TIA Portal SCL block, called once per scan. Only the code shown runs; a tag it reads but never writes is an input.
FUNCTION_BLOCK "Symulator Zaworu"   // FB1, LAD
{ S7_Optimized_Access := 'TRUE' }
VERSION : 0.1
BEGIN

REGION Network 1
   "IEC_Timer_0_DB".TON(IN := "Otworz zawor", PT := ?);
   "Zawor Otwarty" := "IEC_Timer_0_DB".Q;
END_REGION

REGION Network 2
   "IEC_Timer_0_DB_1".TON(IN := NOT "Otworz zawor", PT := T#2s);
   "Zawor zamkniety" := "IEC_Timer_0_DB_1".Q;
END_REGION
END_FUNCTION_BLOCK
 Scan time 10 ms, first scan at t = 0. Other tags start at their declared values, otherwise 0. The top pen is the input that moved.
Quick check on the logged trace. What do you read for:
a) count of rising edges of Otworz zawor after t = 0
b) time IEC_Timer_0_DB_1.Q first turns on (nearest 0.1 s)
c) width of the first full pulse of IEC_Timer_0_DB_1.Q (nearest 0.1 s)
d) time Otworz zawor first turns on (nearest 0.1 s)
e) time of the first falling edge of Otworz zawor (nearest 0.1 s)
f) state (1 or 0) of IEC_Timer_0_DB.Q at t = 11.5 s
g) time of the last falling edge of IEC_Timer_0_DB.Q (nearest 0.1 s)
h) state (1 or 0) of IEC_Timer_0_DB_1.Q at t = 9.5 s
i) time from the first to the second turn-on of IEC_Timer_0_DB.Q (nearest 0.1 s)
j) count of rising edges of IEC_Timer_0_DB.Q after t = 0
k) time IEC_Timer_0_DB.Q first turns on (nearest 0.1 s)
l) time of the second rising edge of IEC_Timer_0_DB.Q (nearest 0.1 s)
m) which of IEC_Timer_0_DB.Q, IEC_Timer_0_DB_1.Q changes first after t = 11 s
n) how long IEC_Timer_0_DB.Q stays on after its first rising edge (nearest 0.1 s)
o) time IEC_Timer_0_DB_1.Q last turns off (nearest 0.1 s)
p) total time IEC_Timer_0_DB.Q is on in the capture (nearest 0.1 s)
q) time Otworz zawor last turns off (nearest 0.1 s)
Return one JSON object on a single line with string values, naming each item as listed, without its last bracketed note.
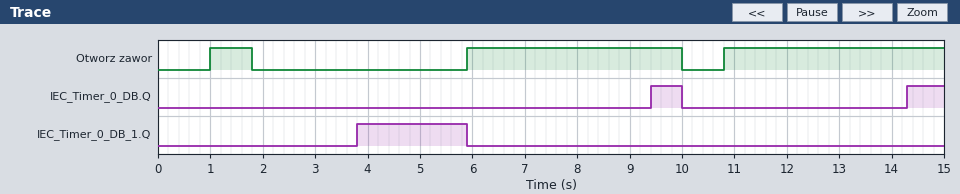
{"count of rising edges of Otworz zawor after t = 0": "3", "time IEC_Timer_0_DB_1.Q first turns on": "3.8 s", "width of the first full pulse of IEC_Timer_0_DB_1.Q": "2.1 s", "time Otworz zawor first turns on": "1.0 s", "time of the first falling edge of Otworz zawor": "1.8 s", "state (1 or 0) of IEC_Timer_0_DB.Q at t = 11.5 s": "0", "time of the last falling edge of IEC_Timer_0_DB.Q": "10.0 s", "state (1 or 0) of IEC_Timer_0_DB_1.Q at t = 9.5 s": "0", "time from the first to the second turn-on of IEC_Timer_0_DB.Q": "4.9 s", "count of rising edges of IEC_Timer_0_DB.Q after t = 0": "2", "time IEC_Timer_0_DB.Q first turns on": "9.4 s", "time of the second rising edge of IEC_Timer_0_DB.Q": "14.3 s", "which of IEC_Timer_0_DB.Q, IEC_Timer_0_DB_1.Q changes first after t = 11 s": "IEC_Timer_0_DB.Q", "how long IEC_Timer_0_DB.Q stays on after its first rising edge": "0.6 s", "time IEC_Timer_0_DB_1.Q last turns off": "5.9 s", "total time IEC_Timer_0_DB.Q is on in the capture": "1.3 s", "time Otworz zawor last turns off": "10.0 s"}
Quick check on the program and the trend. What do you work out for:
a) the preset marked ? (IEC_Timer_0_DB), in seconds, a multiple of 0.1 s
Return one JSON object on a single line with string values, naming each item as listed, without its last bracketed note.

{"the preset marked ? (IEC_Timer_0_DB), in seconds, a multiple of 0.1 s": "3.5 s"}
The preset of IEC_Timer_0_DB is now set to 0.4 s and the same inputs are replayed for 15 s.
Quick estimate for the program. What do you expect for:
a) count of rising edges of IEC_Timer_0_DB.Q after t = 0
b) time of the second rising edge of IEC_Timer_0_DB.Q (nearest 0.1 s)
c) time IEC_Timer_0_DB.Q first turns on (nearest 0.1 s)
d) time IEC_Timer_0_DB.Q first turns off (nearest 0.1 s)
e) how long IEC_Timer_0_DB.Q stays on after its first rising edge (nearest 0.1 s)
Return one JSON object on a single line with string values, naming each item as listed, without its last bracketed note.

{"count of rising edges of IEC_Timer_0_DB.Q after t = 0": "3", "time of the second rising edge of IEC_Timer_0_DB.Q": "6.3 s", "time IEC_Timer_0_DB.Q first turns on": "1.4 s", "time IEC_Timer_0_DB.Q first turns off": "1.8 s", "how long IEC_Timer_0_DB.Q stays on after its first rising edge": "0.4 s"}
